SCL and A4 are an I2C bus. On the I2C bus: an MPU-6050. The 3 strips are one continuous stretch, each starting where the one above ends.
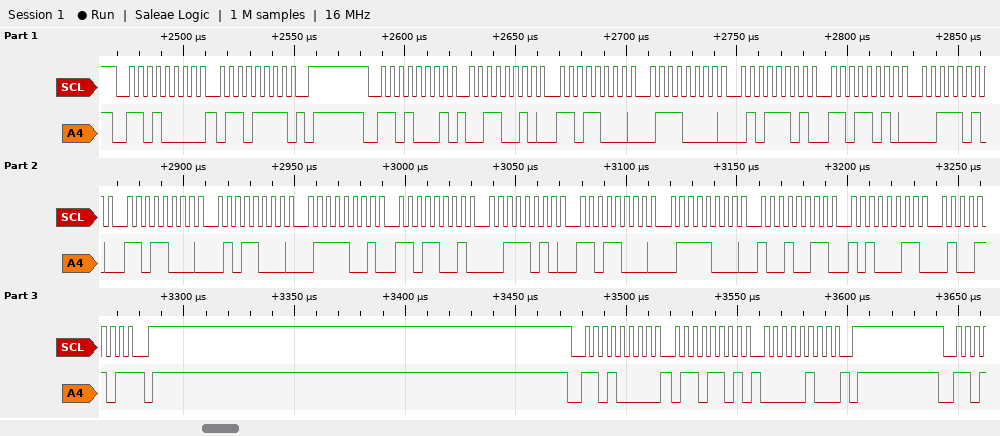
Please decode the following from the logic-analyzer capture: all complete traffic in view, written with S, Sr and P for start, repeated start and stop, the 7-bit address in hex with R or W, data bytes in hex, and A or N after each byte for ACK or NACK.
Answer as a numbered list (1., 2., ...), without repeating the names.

1. S 68W A 6F A P S 68R A 32 A D8 A 70 A 5D A DA A 3A A D8 A 58 A 79 A D9 A 3A A D8 A 78 A 93 A A3 A 4D N P S 68W A 6D A 04 A P
